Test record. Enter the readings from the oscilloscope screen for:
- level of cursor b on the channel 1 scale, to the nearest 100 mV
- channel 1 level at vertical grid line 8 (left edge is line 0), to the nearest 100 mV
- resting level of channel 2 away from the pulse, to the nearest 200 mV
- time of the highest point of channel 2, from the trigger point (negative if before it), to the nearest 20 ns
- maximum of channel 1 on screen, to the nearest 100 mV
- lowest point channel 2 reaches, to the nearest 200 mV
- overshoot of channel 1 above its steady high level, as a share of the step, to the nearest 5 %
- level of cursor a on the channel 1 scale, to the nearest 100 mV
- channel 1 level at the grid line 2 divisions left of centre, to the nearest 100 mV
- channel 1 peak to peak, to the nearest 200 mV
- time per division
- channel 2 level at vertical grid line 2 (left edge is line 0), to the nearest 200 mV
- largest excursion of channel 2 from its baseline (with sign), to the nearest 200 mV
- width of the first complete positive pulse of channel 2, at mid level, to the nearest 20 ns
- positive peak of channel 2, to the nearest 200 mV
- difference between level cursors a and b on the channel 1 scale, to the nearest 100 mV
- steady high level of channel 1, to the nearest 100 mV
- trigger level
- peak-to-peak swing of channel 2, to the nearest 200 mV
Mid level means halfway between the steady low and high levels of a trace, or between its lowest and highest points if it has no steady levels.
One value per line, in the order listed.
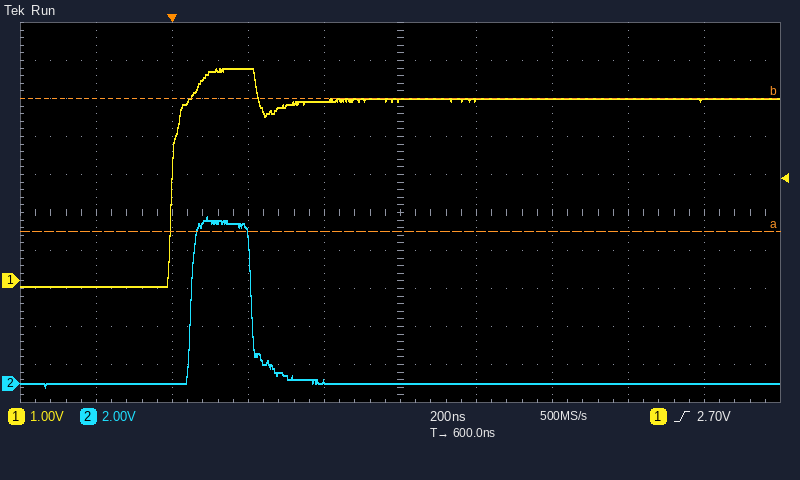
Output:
4.8 V
4.8 V
0.0 V
+100 ns
5.6 V
-200 mV
15 %
1.3 V
5.6 V
5.8 V
200 ns
0.0 V
+8.8 V
160 ns
8.8 V
3.5 V
4.8 V
2.70 V
9.0 V
